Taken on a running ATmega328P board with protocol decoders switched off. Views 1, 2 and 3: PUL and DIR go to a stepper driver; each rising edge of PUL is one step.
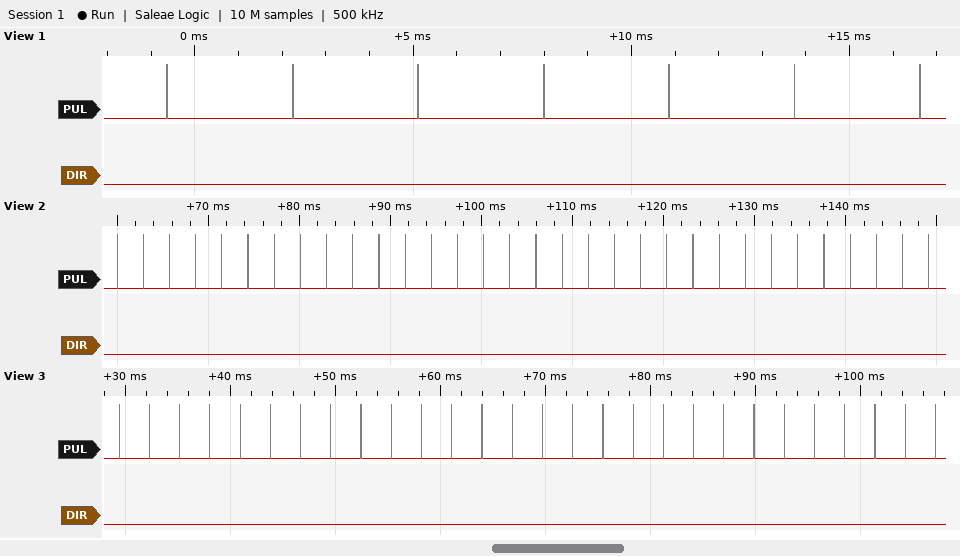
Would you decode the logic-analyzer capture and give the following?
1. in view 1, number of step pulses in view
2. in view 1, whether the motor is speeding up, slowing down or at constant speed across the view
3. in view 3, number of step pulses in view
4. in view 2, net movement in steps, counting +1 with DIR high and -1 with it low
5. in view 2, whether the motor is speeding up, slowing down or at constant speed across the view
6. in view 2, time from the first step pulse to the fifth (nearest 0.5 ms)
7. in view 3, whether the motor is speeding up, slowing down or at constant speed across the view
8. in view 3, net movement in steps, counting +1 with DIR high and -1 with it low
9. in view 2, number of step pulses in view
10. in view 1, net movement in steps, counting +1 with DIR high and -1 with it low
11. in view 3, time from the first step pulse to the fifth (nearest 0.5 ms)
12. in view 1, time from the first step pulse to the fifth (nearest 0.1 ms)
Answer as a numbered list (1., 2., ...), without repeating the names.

1. 7
2. constant speed
3. 28
4. -32
5. constant speed
6. 11.5 ms
7. constant speed
8. -28
9. 32
10. -7
11. 11.5 ms
12. 11.5 ms
